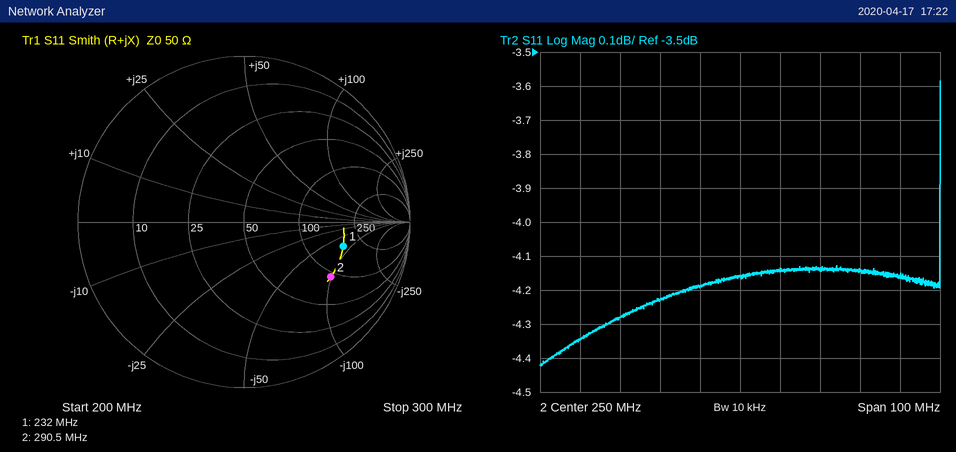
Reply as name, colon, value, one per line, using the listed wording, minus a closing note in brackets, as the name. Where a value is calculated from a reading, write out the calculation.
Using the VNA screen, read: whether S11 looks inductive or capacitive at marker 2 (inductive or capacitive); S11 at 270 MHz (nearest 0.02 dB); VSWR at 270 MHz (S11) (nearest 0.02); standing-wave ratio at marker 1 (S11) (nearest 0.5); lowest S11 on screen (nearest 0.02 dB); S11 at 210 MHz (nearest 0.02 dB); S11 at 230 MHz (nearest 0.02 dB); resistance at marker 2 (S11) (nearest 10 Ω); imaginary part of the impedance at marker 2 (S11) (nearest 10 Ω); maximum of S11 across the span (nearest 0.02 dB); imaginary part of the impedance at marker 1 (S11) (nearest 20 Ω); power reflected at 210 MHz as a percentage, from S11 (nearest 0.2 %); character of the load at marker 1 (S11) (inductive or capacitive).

whether S11 looks inductive or capacitive at marker 2: capacitive
S11 at 270 MHz: -4.14 dB
VSWR at 270 MHz (S11): |Γ| = 10^(-4.14/20) = 0.6209; VSWR = (1 + 0.6209)/(1 − 0.6209) ≈ 4.28
standing-wave ratio at marker 1 (S11): 4.0
lowest S11 on screen: -4.42 dB
S11 at 210 MHz: -4.34 dB
S11 at 230 MHz: -4.22 dB
resistance at marker 2 (S11): 90 Ω
imaginary part of the impedance at marker 2 (S11): -100 Ω
maximum of S11 across the span: -3.58 dB
imaginary part of the impedance at marker 1 (S11): -80 Ω
power reflected at 210 MHz as a percentage, from S11: 10^(-4.34/10) ≈ 36.8 %
character of the load at marker 1 (S11): capacitive
